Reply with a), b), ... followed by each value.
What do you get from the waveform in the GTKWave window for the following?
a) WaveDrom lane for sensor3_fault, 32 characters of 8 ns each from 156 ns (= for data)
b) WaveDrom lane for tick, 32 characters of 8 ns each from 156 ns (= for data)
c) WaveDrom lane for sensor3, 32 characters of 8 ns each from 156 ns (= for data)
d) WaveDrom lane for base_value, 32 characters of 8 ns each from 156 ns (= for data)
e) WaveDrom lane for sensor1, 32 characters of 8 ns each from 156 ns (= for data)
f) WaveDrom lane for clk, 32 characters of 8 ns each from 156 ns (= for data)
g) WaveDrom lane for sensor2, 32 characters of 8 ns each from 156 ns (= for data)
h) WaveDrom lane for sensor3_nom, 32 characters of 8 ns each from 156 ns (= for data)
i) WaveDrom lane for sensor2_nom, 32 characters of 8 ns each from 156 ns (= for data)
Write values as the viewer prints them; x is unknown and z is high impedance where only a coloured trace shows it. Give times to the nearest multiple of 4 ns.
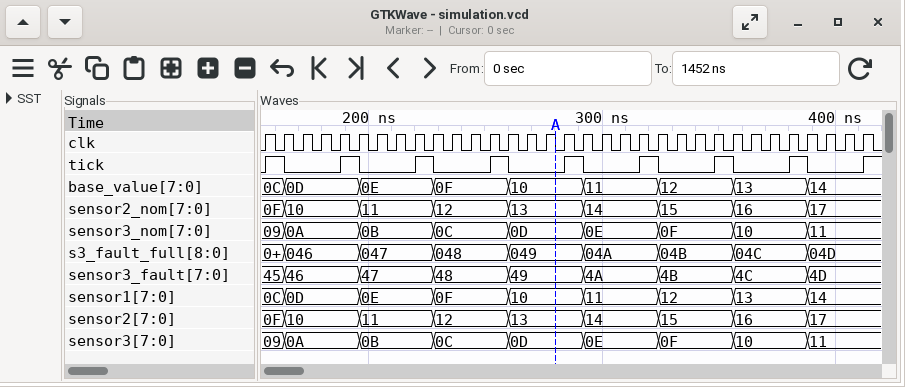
a) {name: 'sensor3_fault', wave: '==...=...=...=...=...=...=...=..', data: '45 46 47 48 49 4A 4B 4C 4D'}
b) {name: 'tick', wave: '10..10..10..10..10..10..10..10..'}
c) {name: 'sensor3', wave: '==...=...=...=...=...=...=...=..', data: '09 0A 0B 0C 0D 0E 0F 10 11'}
d) {name: 'base_value', wave: '==...=...=...=...=...=...=...=..', data: '0C 0D 0E 0F 10 11 12 13 14'}
e) {name: 'sensor1', wave: '==...=...=...=...=...=...=...=..', data: '0C 0D 0E 0F 10 11 12 13 14'}
f) {name: 'clk', wave: 'p...............................'}
g) {name: 'sensor2', wave: '==...=...=...=...=...=...=...=..', data: '0F 10 11 12 13 14 15 16 17'}
h) {name: 'sensor3_nom', wave: '==...=...=...=...=...=...=...=..', data: '09 0A 0B 0C 0D 0E 0F 10 11'}
i) {name: 'sensor2_nom', wave: '==...=...=...=...=...=...=...=..', data: '0F 10 11 12 13 14 15 16 17'}
